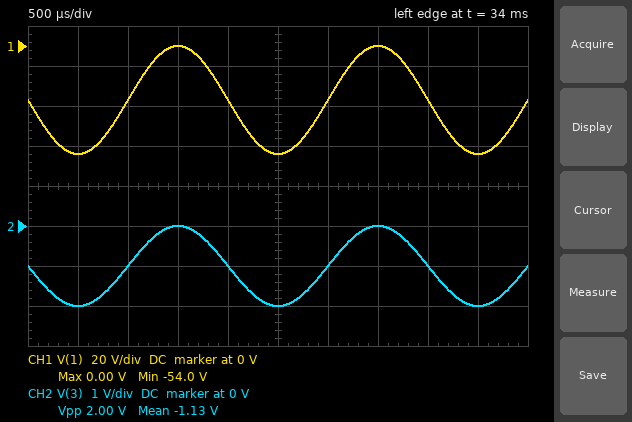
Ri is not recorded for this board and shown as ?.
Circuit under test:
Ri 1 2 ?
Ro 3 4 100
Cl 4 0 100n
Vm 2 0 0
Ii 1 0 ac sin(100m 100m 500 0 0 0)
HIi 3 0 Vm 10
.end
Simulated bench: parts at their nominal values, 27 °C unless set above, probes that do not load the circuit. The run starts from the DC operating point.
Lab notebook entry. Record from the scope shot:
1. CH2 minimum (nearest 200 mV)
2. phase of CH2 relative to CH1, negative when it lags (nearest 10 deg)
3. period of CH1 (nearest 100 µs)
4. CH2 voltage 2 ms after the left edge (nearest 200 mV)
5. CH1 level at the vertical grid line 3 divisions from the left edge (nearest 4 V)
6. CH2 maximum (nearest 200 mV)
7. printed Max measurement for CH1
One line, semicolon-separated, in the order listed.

-2.0 V; 0 deg; 2.0 ms; -1.0 V; 0 V; 0 V; 0.00 V
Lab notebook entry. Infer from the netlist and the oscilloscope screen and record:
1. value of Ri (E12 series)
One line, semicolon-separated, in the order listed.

270 Ω
